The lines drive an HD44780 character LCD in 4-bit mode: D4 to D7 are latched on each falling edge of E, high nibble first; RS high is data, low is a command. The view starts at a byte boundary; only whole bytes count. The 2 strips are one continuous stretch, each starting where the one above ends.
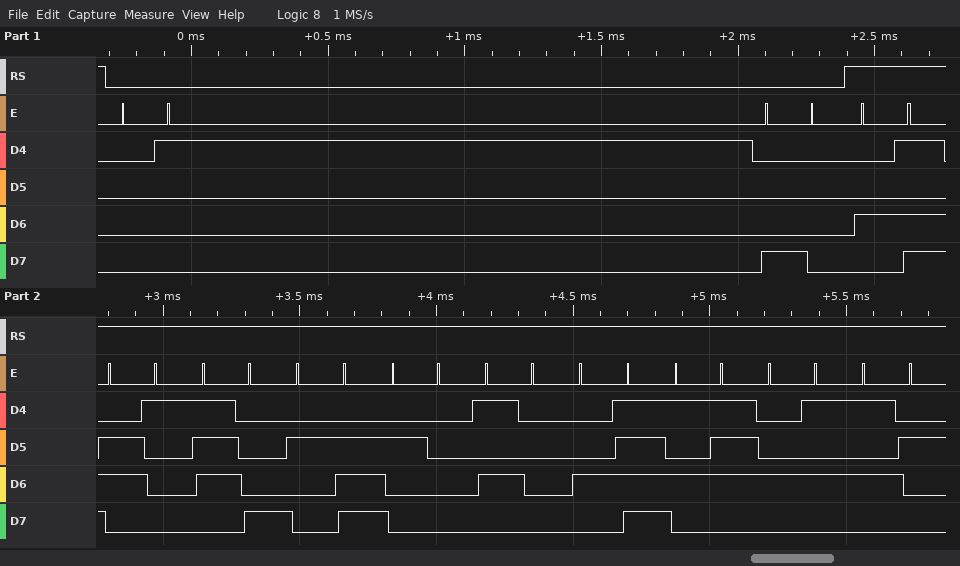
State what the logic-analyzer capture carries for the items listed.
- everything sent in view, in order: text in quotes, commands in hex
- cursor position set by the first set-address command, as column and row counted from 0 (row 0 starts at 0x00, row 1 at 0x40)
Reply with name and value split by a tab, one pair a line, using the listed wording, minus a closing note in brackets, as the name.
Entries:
everything sent in view, in order: text in quotes, commands in hex	0x01 0x80 "Max. POWER"
cursor position set by the first set-address command, as column and row counted from 0	column 0, row 0
